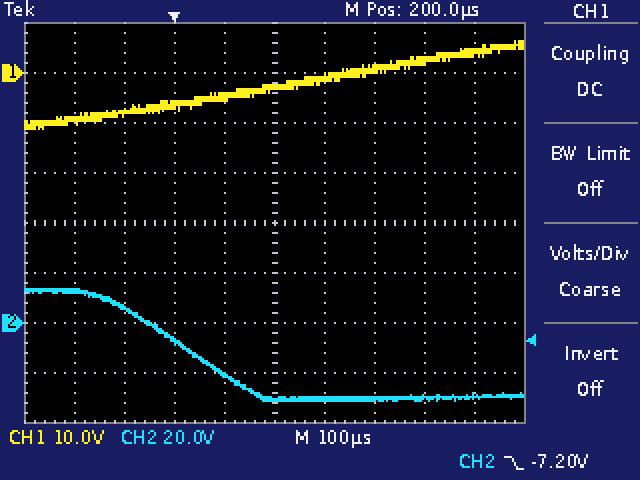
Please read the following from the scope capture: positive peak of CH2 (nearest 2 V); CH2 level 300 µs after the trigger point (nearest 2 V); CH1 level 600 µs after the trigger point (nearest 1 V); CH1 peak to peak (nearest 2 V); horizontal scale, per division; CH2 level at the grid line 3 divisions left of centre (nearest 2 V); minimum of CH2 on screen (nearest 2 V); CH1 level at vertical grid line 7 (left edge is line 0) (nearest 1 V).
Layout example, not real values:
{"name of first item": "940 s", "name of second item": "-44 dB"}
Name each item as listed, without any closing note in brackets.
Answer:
{"positive peak of CH2": "14 V", "CH2 level 300 µs after the trigger point": "-30 V", "CH1 level 600 µs after the trigger point": "4 V", "CH1 peak to peak": "18 V", "horizontal scale, per division": "100 µs", "CH2 level at the grid line 3 divisions left of centre": "6 V", "minimum of CH2 on screen": "-32 V", "CH1 level at vertical grid line 7 (left edge is line 0)": "1 V"}
